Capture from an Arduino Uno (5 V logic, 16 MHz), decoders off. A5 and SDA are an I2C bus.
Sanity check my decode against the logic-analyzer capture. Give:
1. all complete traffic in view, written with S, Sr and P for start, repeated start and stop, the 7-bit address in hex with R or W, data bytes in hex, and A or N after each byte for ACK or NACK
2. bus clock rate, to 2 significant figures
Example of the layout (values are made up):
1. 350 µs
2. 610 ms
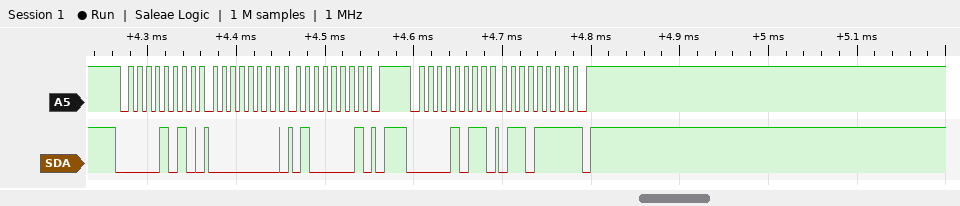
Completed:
1. S 05W A 00 A 41 A P S 05R A 6F N P
2. 100 kHz
